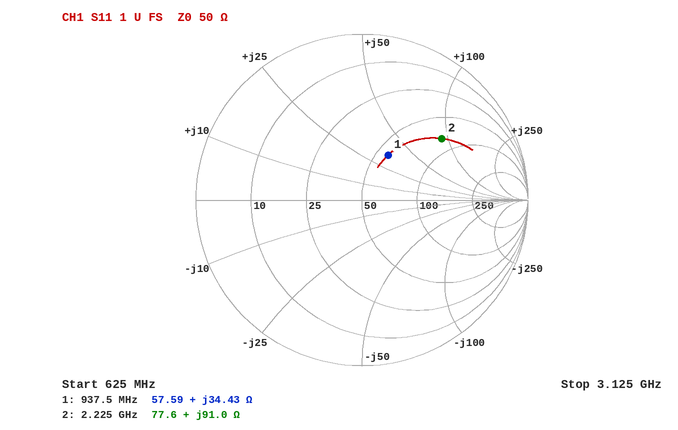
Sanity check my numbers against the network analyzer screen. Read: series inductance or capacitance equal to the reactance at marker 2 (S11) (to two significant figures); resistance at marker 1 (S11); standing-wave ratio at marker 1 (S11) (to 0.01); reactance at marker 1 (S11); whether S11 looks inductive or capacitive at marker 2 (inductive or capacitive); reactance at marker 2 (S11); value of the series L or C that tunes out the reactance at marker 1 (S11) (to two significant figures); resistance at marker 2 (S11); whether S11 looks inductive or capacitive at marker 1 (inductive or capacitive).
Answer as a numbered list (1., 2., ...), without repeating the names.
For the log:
1. 6.5 nH
2. 57.59 Ω
3. 1.91
4. +34.43 Ω
5. inductive
6. +91.0 Ω
7. 4.9 pF
8. 77.6 Ω
9. inductive
